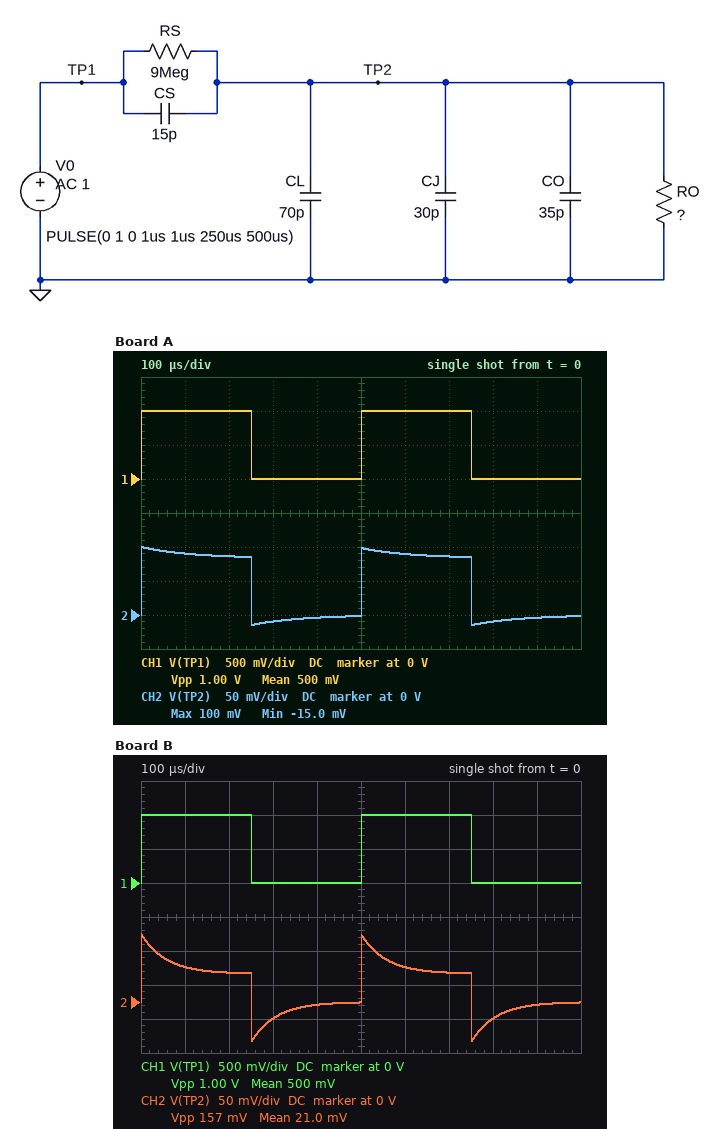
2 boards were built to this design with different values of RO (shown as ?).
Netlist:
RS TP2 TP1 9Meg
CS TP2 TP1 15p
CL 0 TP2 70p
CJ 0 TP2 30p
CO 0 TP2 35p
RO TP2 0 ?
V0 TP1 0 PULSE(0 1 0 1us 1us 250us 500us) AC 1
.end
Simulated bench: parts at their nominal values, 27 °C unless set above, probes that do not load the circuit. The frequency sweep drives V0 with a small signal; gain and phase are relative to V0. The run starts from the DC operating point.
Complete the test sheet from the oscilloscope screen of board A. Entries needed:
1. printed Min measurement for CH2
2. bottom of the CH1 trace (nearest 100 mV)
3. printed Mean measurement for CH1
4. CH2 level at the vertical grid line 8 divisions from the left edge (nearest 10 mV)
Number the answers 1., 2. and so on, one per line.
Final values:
1. -15.0 mV
2. 0 V
3. 500 mV
4. -10 mV
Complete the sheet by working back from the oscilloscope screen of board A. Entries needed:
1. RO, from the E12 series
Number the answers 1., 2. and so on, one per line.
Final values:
1. 820 kΩ
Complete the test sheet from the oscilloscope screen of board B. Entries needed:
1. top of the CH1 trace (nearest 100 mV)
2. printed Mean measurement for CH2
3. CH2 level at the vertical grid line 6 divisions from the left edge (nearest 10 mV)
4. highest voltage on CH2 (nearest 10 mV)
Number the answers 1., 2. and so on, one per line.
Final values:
1. 1.0 V
2. 21.0 mV
3. 50 mV
4. 100 mV
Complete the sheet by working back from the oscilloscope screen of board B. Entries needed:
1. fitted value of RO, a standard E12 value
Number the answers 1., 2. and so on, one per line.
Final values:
1. 390 kΩ
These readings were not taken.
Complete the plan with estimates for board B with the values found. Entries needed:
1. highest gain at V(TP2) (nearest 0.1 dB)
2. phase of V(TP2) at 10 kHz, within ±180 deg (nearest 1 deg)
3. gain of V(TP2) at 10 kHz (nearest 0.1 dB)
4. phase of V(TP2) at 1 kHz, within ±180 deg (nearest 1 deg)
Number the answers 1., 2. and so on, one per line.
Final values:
1. -20.0 dB
2. 9 deg
3. -20.3 dB
4. 21 deg
